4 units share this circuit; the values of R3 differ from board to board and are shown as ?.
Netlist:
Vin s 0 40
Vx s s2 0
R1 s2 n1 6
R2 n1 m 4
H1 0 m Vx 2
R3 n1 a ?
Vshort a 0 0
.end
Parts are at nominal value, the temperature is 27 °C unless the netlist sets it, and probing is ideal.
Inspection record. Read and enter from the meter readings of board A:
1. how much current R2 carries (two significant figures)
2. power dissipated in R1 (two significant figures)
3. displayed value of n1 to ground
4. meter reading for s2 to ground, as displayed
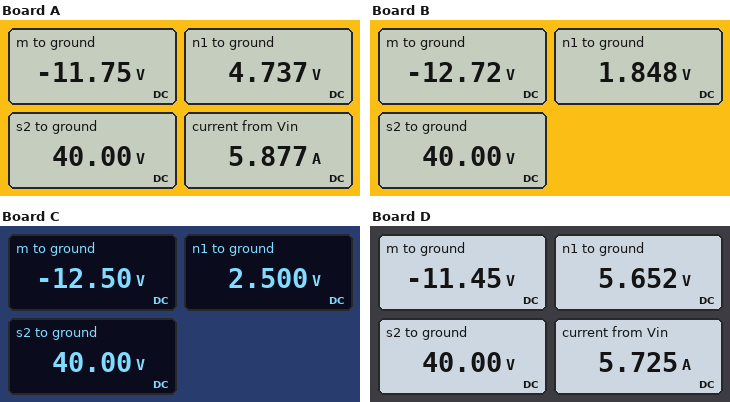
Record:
4.1 A
210 W
4.737 V
40.00 V
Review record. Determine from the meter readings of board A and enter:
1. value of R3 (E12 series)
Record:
2.7 Ω
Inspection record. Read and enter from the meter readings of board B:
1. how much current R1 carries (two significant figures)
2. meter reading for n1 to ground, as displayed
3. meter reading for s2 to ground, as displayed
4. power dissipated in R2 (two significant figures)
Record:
6.4 A
1.848 V
40.00 V
53 W
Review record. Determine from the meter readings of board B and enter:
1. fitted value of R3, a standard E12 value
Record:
0.68 Ω
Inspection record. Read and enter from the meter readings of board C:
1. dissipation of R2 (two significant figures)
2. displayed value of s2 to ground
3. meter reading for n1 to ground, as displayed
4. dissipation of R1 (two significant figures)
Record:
56 W
40.00 V
2.500 V
230 W
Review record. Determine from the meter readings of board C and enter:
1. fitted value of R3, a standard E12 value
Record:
1 Ω
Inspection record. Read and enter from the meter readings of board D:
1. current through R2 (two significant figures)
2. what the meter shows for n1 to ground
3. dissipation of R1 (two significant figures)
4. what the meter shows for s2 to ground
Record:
4.3 A
5.652 V
200 W
40.00 V
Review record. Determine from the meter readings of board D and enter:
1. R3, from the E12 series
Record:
3.9 Ω
